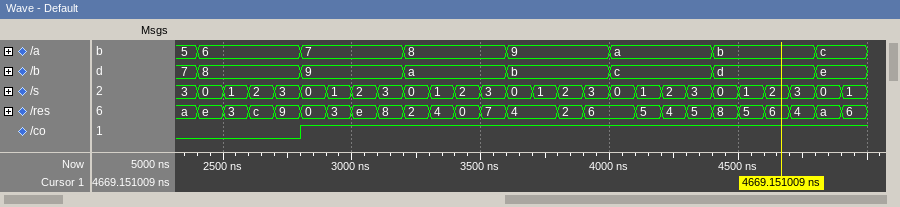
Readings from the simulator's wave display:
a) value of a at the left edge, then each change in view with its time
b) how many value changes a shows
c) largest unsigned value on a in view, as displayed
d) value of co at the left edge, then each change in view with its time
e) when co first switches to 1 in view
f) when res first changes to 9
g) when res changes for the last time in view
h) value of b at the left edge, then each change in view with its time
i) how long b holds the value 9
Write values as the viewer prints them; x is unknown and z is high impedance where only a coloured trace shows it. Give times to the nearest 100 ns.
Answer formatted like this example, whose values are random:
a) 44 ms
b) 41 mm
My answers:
a) 5, 6 at 2400 ns, 7 at 2800 ns, 8 at 3200 ns, 9 at 3600 ns, a at 4000 ns, b at 4400 ns, c at 4800 ns
b) 7
c) c
d) 0, 1 at 2800 ns
e) 2800 ns
f) 2700 ns
g) 4900 ns
h) 7, 8 at 2400 ns, 9 at 2800 ns, a at 3200 ns, b at 3600 ns, c at 4000 ns, d at 4400 ns, e at 4800 ns
i) 400 ns
